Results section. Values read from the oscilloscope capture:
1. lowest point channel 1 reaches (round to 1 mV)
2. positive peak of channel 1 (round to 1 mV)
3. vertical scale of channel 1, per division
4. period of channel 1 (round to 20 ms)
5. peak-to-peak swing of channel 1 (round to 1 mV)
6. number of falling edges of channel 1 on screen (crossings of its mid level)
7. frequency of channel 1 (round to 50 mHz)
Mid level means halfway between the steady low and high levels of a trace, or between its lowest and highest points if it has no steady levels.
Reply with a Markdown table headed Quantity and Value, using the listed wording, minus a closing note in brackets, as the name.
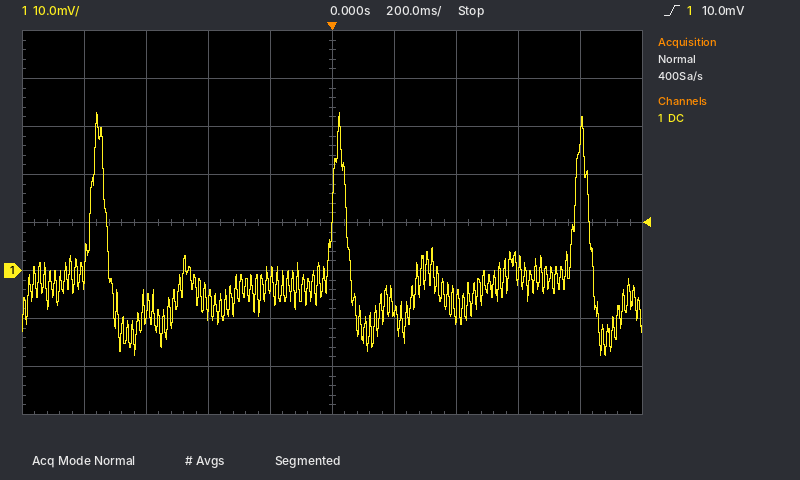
| Quantity | Value |
|---|---|
| lowest point channel 1 reaches | -18 mV |
| positive peak of channel 1 | 33 mV |
| vertical scale of channel 1, per division | 10 mV |
| period of channel 1 | 780 ms |
| peak-to-peak swing of channel 1 | 51 mV |
| number of falling edges of channel 1 on screen | 3 |
| frequency of channel 1 | 1.30 Hz |
